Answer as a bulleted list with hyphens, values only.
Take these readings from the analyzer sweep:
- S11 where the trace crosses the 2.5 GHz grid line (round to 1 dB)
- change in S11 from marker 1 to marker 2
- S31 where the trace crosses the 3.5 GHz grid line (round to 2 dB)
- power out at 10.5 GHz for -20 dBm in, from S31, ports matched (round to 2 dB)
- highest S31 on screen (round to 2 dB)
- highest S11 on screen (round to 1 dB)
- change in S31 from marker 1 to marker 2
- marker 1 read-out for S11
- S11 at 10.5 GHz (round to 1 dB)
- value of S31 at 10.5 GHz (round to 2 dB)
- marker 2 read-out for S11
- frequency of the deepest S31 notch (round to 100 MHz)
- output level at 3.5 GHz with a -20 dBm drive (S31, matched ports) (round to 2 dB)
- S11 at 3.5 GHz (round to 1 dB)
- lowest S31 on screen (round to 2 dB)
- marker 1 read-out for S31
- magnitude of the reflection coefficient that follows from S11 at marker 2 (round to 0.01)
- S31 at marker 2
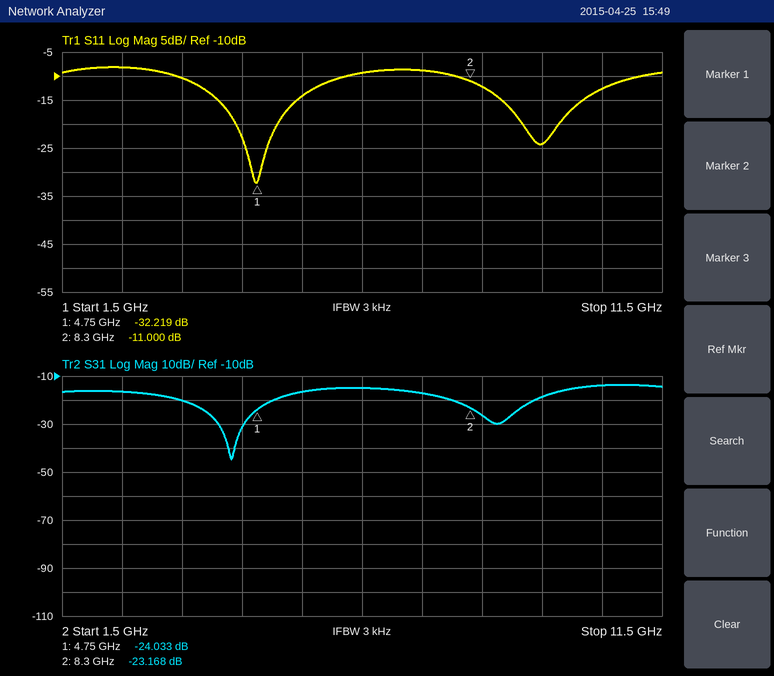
- -8 dB
- 21.219 dB
- -20 dB
- -34 dBm
- -14 dB
- -8 dB
- 0.865 dB
- -32.219 dB
- -13 dB
- -14 dB
- -11.000 dB
- 4.3 GHz
- -40 dBm
- -10 dB
- -44 dB
- -24.033 dB
- 0.28
- -23.168 dB
